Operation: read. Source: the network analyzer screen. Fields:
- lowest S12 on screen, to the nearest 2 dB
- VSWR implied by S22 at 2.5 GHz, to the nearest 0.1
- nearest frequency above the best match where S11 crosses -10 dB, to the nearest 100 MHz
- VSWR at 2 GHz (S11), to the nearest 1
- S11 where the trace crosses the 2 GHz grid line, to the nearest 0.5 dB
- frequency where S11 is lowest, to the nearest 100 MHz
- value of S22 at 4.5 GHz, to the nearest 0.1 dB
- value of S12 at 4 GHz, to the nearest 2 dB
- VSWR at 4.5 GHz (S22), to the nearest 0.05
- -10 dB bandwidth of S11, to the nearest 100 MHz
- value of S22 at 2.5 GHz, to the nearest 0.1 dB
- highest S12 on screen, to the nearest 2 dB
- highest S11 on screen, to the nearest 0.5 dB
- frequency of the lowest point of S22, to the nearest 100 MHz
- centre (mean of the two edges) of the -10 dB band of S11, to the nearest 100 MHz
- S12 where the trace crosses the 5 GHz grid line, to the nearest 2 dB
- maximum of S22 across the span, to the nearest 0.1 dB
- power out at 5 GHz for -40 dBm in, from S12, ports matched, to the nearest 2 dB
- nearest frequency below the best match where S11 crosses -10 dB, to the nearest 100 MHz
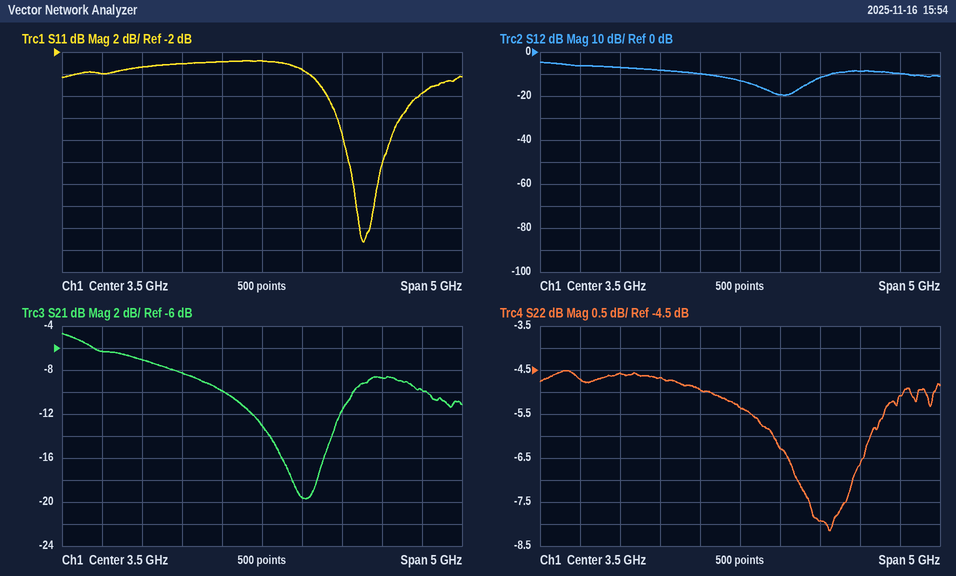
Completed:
-20 dB
3.8
5.1 GHz
5
-3.5 dB
4.8 GHz
-7.9 dB
-20 dB
2.35
600 MHz
-4.7 dB
-4 dB
-3.0 dB
4.6 GHz
4.8 GHz
-8 dB
-4.5 dB
-48 dBm
4.5 GHz
